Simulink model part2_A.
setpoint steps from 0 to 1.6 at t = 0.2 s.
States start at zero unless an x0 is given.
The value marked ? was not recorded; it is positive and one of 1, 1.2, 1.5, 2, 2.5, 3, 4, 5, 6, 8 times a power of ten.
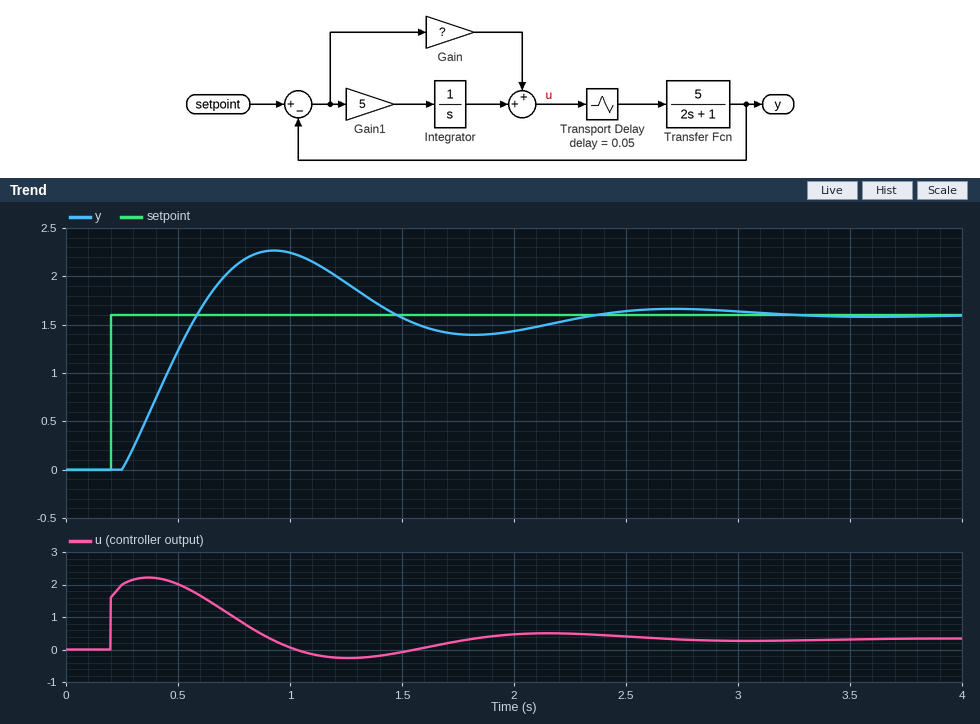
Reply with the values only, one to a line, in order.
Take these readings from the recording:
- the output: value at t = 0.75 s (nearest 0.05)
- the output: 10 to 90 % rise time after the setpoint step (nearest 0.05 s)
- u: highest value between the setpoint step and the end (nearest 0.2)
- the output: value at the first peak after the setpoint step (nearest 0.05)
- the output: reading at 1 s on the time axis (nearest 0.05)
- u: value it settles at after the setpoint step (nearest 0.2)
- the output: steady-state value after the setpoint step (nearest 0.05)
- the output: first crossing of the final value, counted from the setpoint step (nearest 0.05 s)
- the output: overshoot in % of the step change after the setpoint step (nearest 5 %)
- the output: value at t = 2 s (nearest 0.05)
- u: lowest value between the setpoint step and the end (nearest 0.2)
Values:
2.10
0.25 s
2.2
2.25
2.25
0.4
1.60
0.40 s
40 %
1.45
-0.2
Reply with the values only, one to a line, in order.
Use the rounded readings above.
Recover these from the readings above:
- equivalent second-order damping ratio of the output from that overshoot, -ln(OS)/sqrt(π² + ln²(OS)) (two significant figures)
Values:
0.28
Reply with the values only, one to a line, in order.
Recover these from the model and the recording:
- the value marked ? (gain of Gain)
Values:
1
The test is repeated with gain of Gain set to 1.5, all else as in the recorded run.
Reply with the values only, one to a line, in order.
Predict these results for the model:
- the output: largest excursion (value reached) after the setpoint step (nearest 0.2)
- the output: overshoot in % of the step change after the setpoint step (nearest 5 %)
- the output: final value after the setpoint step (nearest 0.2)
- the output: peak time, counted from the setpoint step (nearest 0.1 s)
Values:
2.0
30 %
1.6
0.6 s
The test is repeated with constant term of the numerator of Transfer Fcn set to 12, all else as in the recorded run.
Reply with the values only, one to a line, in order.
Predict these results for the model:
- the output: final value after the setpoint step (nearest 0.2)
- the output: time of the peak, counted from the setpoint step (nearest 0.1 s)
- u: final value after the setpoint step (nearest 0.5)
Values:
1.6
0.4 s
0.0
